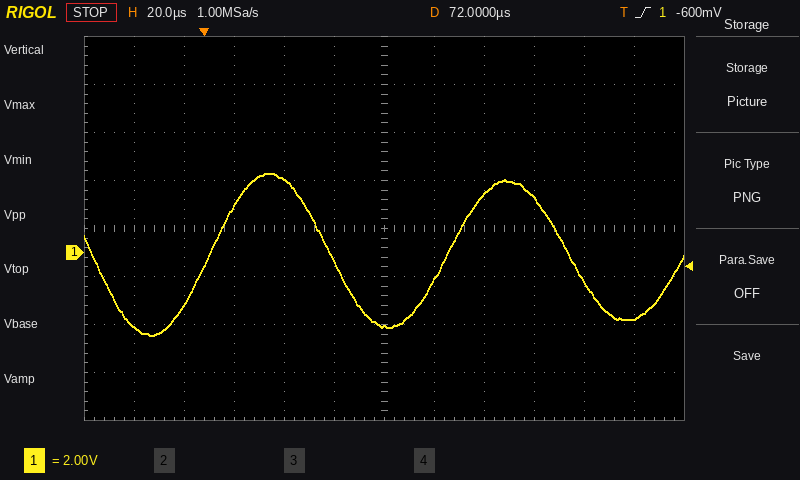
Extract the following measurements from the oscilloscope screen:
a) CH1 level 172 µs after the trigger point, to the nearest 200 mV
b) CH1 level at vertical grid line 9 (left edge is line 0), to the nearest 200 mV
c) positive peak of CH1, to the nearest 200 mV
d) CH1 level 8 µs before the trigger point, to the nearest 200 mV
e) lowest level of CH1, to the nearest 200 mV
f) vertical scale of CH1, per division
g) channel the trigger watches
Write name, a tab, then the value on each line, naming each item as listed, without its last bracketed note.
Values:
CH1 level 172 µs after the trigger point, to the nearest 200 mV	-2.8 V
CH1 level at vertical grid line 9 (left edge is line 0), to the nearest 200 mV	2.2 V
positive peak of CH1, to the nearest 200 mV	3.2 V
CH1 level 8 µs before the trigger point, to the nearest 200 mV	-2.2 V
lowest level of CH1, to the nearest 200 mV	-3.4 V
vertical scale of CH1, per division	2 V
channel the trigger watches	CH1
